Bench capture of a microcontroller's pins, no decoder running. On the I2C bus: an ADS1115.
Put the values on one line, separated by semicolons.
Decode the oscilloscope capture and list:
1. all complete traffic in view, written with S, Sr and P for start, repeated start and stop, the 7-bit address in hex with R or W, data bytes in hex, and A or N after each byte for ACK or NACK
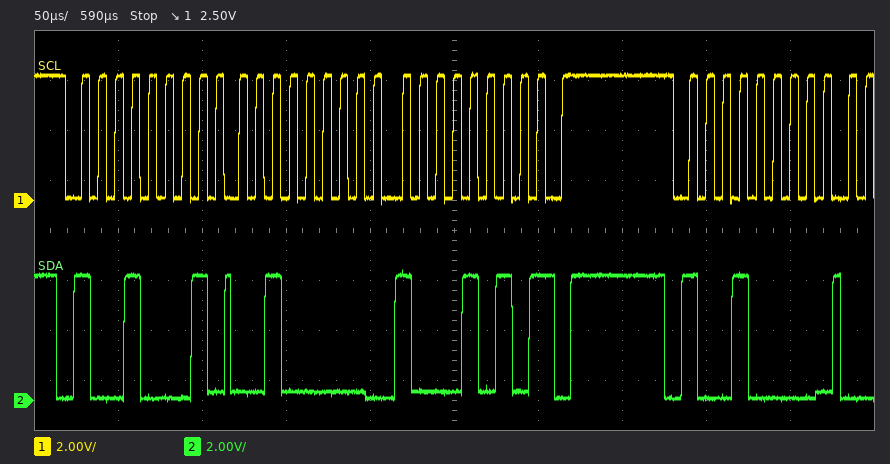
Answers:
S 48R A 20 A 8A N P S 48W A
